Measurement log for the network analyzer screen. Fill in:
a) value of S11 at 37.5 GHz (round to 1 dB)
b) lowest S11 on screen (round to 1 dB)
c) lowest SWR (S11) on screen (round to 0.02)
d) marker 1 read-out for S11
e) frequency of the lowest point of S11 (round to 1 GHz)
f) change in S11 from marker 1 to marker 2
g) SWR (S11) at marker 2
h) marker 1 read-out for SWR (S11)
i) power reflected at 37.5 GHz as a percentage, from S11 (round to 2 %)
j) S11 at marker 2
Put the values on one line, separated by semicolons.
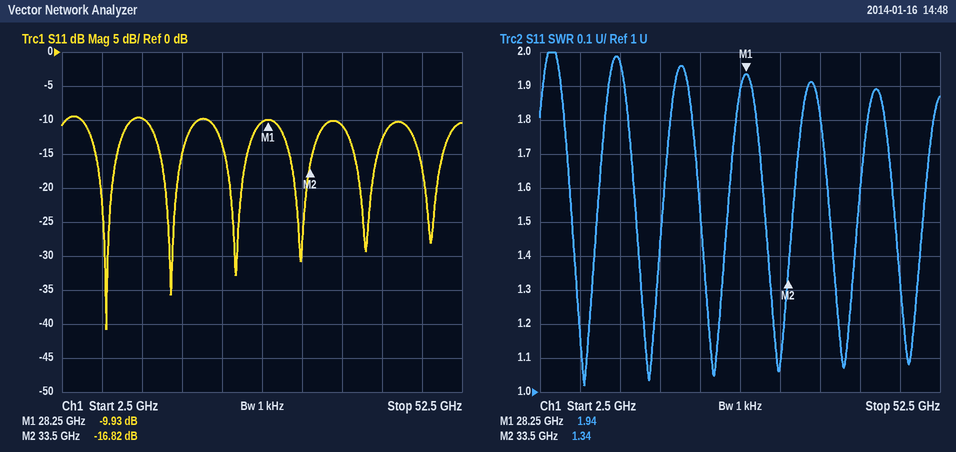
-11 dB; -41 dB; 1.02; -9.93 dB; 8 GHz; -6.89 dB; 1.34; 1.94; 8 %; -16.82 dB
